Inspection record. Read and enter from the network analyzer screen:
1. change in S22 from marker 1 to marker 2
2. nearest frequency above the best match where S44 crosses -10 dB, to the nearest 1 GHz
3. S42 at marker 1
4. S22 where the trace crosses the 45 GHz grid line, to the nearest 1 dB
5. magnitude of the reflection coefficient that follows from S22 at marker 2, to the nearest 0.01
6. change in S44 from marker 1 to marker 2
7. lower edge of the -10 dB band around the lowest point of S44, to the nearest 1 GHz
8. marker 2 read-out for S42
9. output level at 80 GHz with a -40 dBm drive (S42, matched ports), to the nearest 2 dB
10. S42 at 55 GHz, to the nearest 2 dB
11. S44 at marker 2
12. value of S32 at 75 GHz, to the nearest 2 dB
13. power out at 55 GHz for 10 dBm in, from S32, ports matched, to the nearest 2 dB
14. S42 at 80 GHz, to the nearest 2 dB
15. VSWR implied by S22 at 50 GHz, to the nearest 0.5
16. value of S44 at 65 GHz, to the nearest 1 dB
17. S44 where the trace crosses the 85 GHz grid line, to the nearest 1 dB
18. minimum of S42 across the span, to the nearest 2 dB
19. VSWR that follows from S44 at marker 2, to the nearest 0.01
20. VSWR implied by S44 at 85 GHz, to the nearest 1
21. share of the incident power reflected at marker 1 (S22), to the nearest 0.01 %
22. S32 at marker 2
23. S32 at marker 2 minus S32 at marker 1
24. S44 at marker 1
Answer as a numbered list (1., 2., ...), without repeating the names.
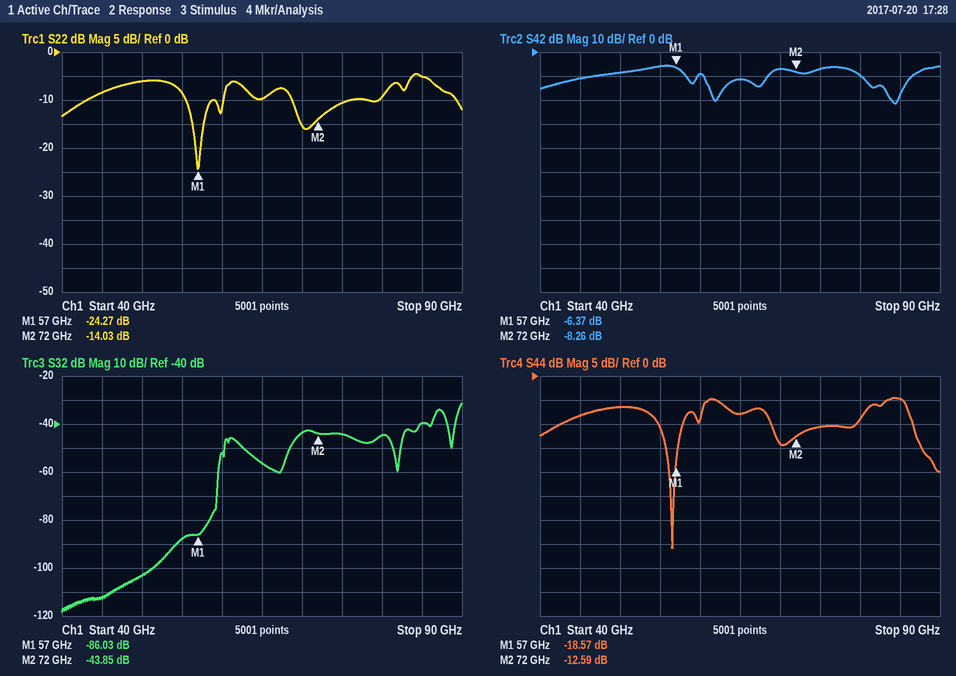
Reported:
1. 10.24 dB
2. 58 GHz
3. -6.37 dB
4. -8 dB
5. 0.20
6. 5.98 dB
7. 55 GHz
8. -8.26 dB
9. -50 dBm
10. -6 dB
11. -12.59 dB
12. -44 dB
13. -78 dBm
14. -10 dB
15. 3.0
16. -8 dB
17. -5 dB
18. -22 dB
19. 1.61
20. 4
21. 0.37 %
22. -43.85 dB
23. 42.18 dB
24. -18.57 dB
